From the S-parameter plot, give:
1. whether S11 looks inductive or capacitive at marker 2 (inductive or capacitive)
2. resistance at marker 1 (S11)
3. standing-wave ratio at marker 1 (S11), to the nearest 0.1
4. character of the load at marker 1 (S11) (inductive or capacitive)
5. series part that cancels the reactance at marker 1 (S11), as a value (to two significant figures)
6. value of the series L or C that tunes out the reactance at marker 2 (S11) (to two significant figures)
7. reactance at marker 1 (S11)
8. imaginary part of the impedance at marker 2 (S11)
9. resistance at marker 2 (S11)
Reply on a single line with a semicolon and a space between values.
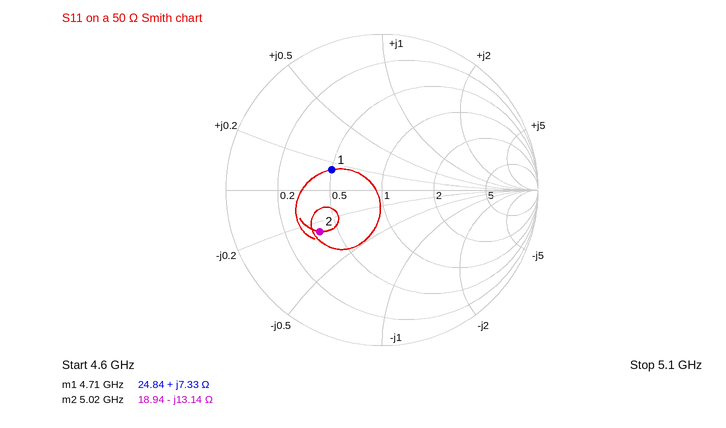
capacitive; 24.84 Ω; 2.1; inductive; 4.6 pF; 420 pH; +7.33 Ω; -13.14 Ω; 18.94 Ω
